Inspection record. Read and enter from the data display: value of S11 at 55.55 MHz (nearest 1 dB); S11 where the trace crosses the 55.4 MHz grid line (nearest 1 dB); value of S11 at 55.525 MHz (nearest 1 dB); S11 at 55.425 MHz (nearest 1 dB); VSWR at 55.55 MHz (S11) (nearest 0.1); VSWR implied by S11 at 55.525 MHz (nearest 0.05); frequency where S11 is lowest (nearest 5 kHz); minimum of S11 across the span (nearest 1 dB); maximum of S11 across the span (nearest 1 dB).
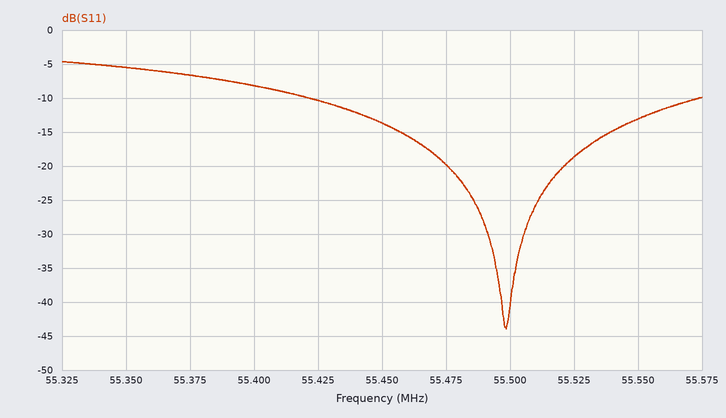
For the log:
-13 dB
-8 dB
-19 dB
-10 dB
1.6
1.25
55.500 MHz
-44 dB
-5 dB
